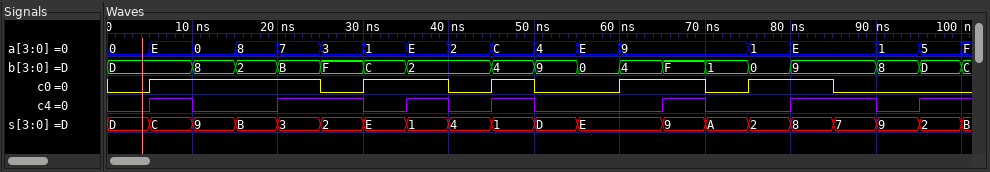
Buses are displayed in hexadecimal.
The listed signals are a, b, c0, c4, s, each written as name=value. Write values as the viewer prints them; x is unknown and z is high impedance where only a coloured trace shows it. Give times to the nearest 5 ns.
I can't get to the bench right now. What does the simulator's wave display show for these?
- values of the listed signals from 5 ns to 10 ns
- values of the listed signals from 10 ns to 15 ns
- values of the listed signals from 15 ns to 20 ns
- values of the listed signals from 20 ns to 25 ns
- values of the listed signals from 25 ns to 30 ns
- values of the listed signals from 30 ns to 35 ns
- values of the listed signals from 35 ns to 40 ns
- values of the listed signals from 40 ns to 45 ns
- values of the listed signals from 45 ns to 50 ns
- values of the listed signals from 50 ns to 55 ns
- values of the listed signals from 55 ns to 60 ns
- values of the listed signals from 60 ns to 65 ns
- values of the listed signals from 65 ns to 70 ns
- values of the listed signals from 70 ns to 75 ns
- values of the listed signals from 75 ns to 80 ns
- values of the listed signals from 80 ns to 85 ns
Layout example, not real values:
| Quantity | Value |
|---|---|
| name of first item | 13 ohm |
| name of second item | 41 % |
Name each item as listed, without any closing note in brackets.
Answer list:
| Quantity | Value |
|---|---|
| values of the listed signals from 5 ns to 10 ns | a=E, b=D, c0=1, c4=1, s=C |
| values of the listed signals from 10 ns to 15 ns | a=0, b=8, c0=1, c4=0, s=9 |
| values of the listed signals from 15 ns to 20 ns | a=8, b=2, c0=1, c4=0, s=B |
| values of the listed signals from 20 ns to 25 ns | a=7, b=B, c0=1, c4=1, s=3 |
| values of the listed signals from 25 ns to 30 ns | a=3, b=F, c0=0, c4=1, s=2 |
| values of the listed signals from 30 ns to 35 ns | a=1, b=C, c0=1, c4=0, s=E |
| values of the listed signals from 35 ns to 40 ns | a=E, b=2, c0=1, c4=1, s=1 |
| values of the listed signals from 40 ns to 45 ns | a=2, b=2, c0=0, c4=0, s=4 |
| values of the listed signals from 45 ns to 50 ns | a=C, b=4, c0=1, c4=1, s=1 |
| values of the listed signals from 50 ns to 55 ns | a=4, b=9, c0=0, c4=0, s=D |
| values of the listed signals from 55 ns to 60 ns | a=E, b=0, c0=0, c4=0, s=E |
| values of the listed signals from 60 ns to 65 ns | a=9, b=4, c0=1, c4=0, s=E |
| values of the listed signals from 65 ns to 70 ns | a=9, b=F, c0=1, c4=1, s=9 |
| values of the listed signals from 70 ns to 75 ns | a=9, b=1, c0=0, c4=0, s=A |
| values of the listed signals from 75 ns to 80 ns | a=1, b=0, c0=1, c4=0, s=2 |
| values of the listed signals from 80 ns to 85 ns | a=E, b=9, c0=1, c4=1, s=8 |
